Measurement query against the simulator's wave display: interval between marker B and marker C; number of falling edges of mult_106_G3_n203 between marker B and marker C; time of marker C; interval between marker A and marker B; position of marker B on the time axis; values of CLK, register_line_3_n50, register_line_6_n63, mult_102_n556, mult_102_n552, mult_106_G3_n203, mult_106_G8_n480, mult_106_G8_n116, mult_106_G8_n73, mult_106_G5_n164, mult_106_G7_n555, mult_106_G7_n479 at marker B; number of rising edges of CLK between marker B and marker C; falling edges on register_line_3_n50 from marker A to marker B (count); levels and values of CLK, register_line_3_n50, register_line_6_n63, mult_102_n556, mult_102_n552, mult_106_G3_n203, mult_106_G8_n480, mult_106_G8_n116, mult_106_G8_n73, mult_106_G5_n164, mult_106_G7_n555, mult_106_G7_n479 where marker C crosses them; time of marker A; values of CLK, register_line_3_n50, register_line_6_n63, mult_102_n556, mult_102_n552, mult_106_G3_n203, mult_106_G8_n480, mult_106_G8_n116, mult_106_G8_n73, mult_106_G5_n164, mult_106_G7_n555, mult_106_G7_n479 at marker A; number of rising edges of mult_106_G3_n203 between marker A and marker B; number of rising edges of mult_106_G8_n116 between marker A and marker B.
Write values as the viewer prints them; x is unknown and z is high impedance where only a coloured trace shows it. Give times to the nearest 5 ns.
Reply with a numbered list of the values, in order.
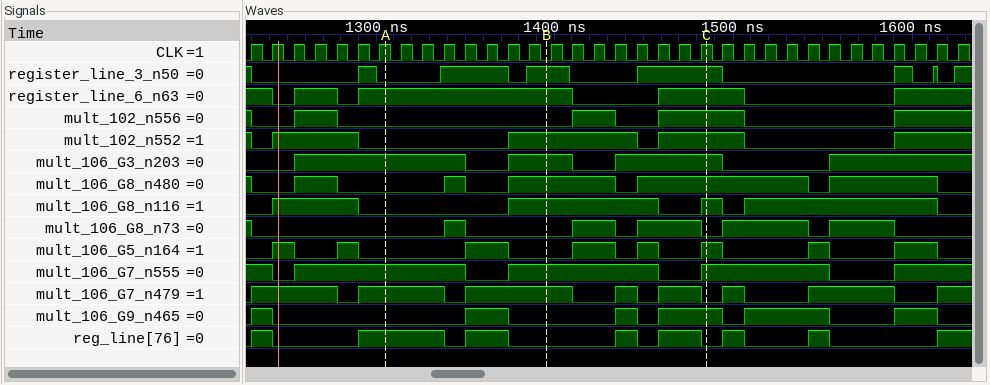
1. 90 ns
2. 1
3. 1485 ns
4. 90 ns
5. 1395 ns
6. CLK=0, register_line_3_n50=1, register_line_6_n63=1, mult_102_n556=0, mult_102_n552=1, mult_106_G3_n203=1, mult_106_G8_n480=1, mult_106_G8_n116=1, mult_106_G8_n73=0, mult_106_G5_n164=0, mult_106_G7_n555=1, mult_106_G7_n479=1
7. 8
8. 1
9. CLK=1, register_line_3_n50=1, register_line_6_n63=1, mult_102_n556=1, mult_102_n552=1, mult_106_G3_n203=1, mult_106_G8_n480=1, mult_106_G8_n116=1, mult_106_G8_n73=0, mult_106_G5_n164=1, mult_106_G7_n555=1, mult_106_G7_n479=0
10. 1305 ns
11. CLK=1, register_line_3_n50=0, register_line_6_n63=1, mult_102_n556=0, mult_102_n552=0, mult_106_G3_n203=1, mult_106_G8_n480=0, mult_106_G8_n116=0, mult_106_G8_n73=0, mult_106_G5_n164=0, mult_106_G7_n555=1, mult_106_G7_n479=1
12. 1
13. 1
